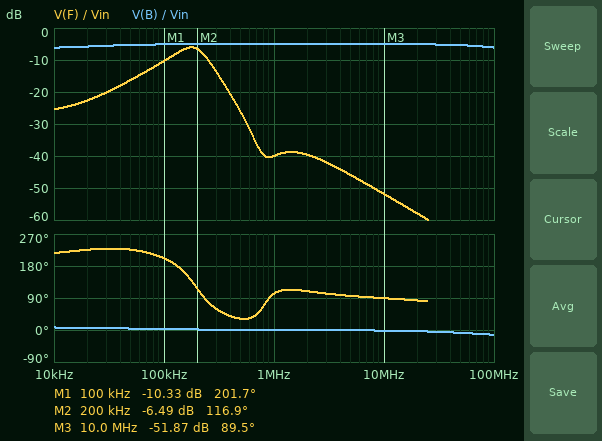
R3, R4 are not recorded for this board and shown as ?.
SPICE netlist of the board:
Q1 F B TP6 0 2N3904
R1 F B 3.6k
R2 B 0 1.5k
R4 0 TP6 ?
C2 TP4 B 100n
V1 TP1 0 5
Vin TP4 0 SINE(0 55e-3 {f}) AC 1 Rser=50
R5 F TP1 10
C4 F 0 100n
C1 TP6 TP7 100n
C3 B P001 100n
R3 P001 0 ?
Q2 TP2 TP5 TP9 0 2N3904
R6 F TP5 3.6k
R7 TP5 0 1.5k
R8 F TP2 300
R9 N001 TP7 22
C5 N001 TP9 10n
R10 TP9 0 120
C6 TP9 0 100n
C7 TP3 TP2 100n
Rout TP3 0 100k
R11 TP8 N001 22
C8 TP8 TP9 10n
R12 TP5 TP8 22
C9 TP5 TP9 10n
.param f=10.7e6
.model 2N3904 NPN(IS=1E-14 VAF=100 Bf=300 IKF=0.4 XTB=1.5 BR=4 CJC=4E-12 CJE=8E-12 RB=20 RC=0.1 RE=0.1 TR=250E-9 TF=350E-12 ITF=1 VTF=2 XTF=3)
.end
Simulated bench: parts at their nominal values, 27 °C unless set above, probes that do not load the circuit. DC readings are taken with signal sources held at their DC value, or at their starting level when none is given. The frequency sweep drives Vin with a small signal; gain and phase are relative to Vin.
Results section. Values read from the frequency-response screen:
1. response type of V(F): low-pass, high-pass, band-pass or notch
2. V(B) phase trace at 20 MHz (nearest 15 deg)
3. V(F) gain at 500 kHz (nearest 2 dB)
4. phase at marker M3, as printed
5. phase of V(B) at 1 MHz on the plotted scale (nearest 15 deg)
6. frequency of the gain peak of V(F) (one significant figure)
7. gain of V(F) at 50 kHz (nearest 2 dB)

band-pass
0 deg
-26 dB
89.5 deg
0 deg
200 kHz
-16 dB
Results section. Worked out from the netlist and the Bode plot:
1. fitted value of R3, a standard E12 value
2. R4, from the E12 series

68 Ω
390 Ω
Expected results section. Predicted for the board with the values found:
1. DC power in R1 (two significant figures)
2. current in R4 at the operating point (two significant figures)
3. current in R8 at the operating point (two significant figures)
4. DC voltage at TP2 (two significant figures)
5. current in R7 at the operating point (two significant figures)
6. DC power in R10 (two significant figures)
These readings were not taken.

3.3 mW
2.0 mA
6.0 mA
3.1 V
950 µA
4.3 mW
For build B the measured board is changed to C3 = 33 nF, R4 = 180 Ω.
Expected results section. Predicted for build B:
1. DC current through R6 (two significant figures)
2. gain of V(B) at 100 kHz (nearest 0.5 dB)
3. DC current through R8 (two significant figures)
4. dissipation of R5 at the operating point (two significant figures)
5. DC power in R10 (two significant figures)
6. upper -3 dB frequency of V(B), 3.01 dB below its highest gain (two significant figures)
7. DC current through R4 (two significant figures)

960 µA
-4.5 dB
5.9 mA
1.4 mW
4.2 mW
80 MHz
4.1 mA
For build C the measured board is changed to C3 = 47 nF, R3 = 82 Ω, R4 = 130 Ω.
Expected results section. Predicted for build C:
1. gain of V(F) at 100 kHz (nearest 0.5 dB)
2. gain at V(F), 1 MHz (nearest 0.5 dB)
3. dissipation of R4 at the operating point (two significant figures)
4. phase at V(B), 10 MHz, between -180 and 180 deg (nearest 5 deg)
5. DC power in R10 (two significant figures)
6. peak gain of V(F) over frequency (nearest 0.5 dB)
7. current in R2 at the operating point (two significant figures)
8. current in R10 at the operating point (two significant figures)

-9.5 dB
-35.0 dB
3.9 mW
0 deg
4.2 mW
-5.5 dB
940 µA
5.9 mA
